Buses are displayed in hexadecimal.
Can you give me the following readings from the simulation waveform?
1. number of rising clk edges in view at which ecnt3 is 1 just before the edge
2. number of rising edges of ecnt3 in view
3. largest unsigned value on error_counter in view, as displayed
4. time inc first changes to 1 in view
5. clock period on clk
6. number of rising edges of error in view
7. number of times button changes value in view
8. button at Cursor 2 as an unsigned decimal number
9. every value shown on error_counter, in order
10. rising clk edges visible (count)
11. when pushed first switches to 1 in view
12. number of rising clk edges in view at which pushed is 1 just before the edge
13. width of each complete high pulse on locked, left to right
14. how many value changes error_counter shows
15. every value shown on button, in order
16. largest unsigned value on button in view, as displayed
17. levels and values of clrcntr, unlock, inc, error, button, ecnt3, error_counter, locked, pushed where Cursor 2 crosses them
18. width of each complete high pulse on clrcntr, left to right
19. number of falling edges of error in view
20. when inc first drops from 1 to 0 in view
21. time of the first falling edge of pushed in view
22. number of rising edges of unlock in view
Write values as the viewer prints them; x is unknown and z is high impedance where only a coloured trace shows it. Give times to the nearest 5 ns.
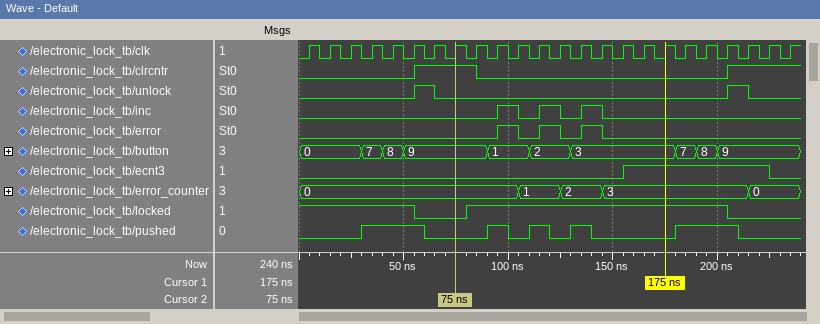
7
1
3
95 ns
10 ns
3
9
9
0, 1, 2, 3, 0
24
30 ns
9
125 ns
4
0, 7, 8, 9, 1, 2, 3, 7, 8, 9
9
clrcntr=1, unlock=0, inc=0, error=0, button=9, ecnt3=0, error_counter=0, locked=0, pushed=0
30 ns
3
105 ns
60 ns
2
